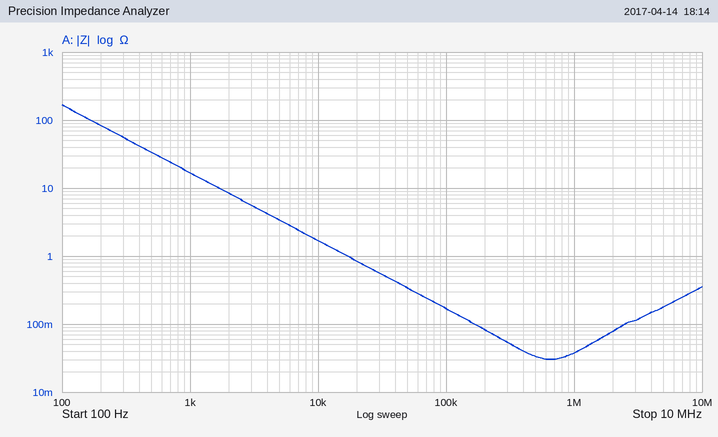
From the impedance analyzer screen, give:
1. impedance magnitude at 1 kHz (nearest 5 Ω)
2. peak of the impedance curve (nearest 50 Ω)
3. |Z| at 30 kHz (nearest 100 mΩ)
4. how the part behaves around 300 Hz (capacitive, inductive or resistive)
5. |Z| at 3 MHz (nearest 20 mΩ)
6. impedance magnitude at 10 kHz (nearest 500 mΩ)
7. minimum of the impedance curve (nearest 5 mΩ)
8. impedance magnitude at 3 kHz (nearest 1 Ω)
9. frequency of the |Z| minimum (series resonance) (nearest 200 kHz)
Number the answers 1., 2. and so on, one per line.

1. 15 Ω
2. 150 Ω
3. 600 mΩ
4. capacitive
5. 120 mΩ
6. 1.5 Ω
7. 30 mΩ
8. 6 Ω
9. 600 kHz
